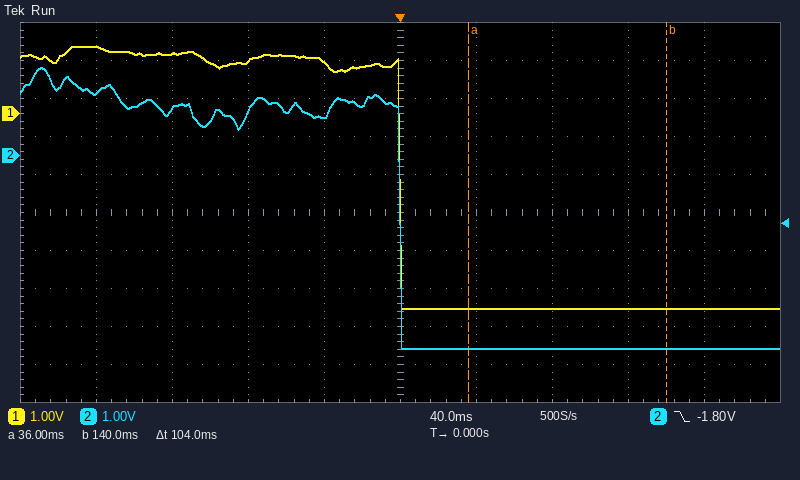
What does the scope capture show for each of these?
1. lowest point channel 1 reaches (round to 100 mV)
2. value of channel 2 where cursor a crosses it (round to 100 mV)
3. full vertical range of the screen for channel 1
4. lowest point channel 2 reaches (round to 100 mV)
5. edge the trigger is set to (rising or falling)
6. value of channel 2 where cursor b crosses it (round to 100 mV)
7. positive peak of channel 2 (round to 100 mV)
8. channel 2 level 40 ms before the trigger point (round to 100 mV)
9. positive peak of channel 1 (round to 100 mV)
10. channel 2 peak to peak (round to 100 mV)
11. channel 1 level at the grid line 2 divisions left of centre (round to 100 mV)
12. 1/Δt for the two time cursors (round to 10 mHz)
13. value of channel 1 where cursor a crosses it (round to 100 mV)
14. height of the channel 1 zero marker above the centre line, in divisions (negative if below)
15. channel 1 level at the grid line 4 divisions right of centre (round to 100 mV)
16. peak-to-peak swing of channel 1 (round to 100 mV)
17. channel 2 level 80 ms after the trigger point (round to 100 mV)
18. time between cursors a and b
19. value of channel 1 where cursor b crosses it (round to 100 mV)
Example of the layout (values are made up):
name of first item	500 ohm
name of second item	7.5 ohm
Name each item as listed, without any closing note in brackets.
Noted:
lowest point channel 1 reaches	-5.1 V
value of channel 2 where cursor a crosses it	-5.1 V
full vertical range of the screen for channel 1	10 V
lowest point channel 2 reaches	-5.1 V
edge the trigger is set to	falling
value of channel 2 where cursor b crosses it	-5.1 V
positive peak of channel 2	2.3 V
channel 2 level 40 ms before the trigger point	1.1 V
positive peak of channel 1	1.8 V
channel 2 peak to peak	7.4 V
channel 1 level at the grid line 2 divisions left of centre	1.4 V
1/Δt for the two time cursors	9.62 Hz
value of channel 1 where cursor a crosses it	-5.1 V
height of the channel 1 zero marker above the centre line, in divisions	+2.6 div
channel 1 level at the grid line 4 divisions right of centre	-5.1 V
peak-to-peak swing of channel 1	6.9 V
channel 2 level 80 ms after the trigger point	-5.1 V
time between cursors a and b	104 ms
value of channel 1 where cursor b crosses it	-5.1 V
